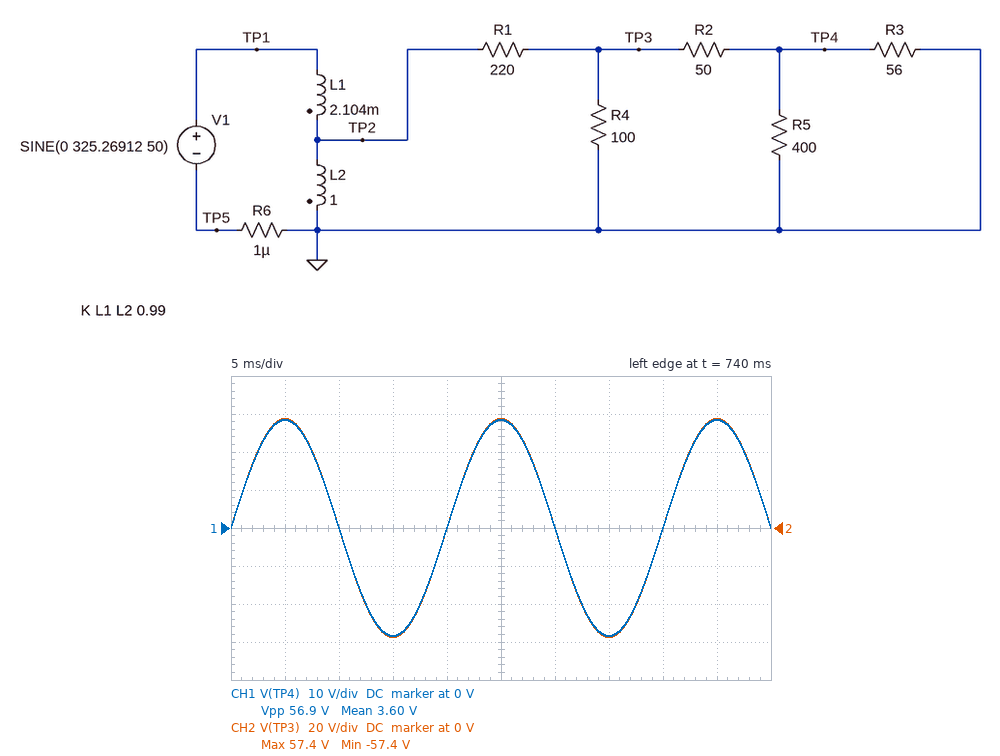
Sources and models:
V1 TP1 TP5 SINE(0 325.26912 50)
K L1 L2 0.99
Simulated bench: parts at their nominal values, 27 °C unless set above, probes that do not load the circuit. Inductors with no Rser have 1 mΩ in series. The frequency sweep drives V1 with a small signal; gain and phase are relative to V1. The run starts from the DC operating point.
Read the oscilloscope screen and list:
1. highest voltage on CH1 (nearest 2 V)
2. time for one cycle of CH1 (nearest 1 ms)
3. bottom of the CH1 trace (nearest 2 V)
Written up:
28 V
20 ms
-28 V
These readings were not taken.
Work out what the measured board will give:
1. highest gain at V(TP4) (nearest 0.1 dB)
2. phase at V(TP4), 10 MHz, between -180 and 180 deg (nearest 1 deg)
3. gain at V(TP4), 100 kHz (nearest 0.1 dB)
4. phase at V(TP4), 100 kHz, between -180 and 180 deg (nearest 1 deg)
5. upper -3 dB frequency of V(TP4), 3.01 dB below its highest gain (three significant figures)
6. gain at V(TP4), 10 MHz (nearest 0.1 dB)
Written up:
-21.2 dB
-84 deg
-21.2 dB
-5 deg
1.12 MHz
-40.2 dB
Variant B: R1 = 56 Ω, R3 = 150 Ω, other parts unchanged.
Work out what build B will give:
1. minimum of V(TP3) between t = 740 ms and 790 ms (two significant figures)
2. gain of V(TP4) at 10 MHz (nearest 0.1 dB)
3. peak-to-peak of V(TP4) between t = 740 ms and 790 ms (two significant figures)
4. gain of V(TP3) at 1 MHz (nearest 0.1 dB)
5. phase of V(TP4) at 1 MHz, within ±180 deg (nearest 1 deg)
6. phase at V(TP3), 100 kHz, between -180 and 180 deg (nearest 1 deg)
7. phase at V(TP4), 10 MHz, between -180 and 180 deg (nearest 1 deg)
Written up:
-160 V
-35.5 dB
220 V
-13.2 dB
-64 deg
-12 deg
-87 deg
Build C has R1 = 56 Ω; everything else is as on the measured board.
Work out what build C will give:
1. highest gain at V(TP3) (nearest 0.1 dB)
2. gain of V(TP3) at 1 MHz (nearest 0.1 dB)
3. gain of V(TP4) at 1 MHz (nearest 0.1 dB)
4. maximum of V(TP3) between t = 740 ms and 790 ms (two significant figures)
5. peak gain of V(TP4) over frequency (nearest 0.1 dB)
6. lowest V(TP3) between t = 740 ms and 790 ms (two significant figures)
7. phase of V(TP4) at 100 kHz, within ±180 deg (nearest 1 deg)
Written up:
-6.9 dB
-14.8 dB
-20.9 dB
150 V
-13.0 dB
-150 V
-13 deg
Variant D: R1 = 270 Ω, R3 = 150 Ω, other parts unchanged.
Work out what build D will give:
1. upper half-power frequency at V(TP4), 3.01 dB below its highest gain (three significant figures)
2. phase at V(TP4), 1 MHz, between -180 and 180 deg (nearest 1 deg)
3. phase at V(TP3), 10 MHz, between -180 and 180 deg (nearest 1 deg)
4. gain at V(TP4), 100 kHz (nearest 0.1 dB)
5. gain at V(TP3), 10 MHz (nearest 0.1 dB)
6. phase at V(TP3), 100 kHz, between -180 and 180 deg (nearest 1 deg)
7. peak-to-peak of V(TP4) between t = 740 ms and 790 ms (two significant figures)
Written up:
1.38 MHz
-36 deg
-82 deg
-18.3 dB
-32.3 dB
-4 deg
79 V
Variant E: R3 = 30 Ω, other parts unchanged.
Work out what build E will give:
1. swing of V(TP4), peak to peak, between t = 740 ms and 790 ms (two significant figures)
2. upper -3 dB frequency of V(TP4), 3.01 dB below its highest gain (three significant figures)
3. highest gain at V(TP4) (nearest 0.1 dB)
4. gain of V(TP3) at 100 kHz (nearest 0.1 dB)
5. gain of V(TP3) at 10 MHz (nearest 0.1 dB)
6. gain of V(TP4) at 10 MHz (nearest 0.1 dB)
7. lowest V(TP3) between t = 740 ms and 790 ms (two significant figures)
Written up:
37 V
1.10 MHz
-24.9 dB
-16.0 dB
-35.2 dB
-44.2 dB
-52 V
